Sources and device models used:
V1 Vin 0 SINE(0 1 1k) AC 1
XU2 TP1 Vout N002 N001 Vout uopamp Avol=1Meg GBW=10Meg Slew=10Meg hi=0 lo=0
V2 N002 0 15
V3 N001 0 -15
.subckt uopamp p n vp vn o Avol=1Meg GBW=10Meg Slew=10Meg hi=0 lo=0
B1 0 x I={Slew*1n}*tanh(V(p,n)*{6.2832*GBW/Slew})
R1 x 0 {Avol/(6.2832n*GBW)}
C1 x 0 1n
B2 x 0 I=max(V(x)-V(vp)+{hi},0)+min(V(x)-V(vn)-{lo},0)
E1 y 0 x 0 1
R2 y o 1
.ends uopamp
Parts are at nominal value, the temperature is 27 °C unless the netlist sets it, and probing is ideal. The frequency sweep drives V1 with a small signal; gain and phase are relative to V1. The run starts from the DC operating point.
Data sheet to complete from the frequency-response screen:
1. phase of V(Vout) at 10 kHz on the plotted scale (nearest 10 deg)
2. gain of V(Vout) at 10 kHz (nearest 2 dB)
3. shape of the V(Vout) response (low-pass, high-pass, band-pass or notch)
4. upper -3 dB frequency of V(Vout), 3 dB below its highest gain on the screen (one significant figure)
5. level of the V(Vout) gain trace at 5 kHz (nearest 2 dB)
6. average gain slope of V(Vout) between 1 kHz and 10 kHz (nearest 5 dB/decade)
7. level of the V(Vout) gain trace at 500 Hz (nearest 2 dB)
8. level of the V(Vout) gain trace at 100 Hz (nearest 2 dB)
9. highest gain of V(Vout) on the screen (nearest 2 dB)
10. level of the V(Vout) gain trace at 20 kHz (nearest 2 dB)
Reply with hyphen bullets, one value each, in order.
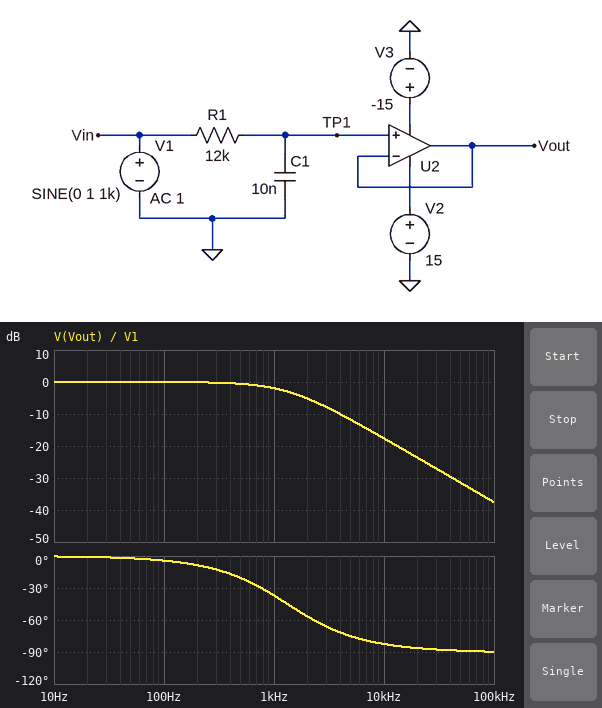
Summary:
- -80 deg
- -18 dB
- low-pass
- 1 kHz
- -12 dB
- -15 dB/decade
- 0 dB
- 0 dB
- 0 dB
- -24 dB
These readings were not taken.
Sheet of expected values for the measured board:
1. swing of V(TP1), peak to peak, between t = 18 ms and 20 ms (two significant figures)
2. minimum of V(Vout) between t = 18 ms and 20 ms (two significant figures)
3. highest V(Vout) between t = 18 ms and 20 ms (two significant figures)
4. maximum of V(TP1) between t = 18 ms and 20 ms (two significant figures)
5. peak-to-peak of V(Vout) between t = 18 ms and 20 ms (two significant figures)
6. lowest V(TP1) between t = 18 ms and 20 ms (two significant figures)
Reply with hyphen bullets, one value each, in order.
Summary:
- 1.6 V
- -800 mV
- 800 mV
- 800 mV
- 1.6 V
- -800 mV
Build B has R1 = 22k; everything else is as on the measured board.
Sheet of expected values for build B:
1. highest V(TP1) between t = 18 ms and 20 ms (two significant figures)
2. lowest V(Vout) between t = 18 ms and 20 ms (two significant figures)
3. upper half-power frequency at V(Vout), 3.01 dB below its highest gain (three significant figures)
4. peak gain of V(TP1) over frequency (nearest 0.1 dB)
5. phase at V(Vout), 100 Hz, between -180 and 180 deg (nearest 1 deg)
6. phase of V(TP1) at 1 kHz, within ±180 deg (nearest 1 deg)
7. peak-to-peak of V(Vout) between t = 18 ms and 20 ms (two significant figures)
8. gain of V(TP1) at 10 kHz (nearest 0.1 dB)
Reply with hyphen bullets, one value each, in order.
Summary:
- 590 mV
- -590 mV
- 723 Hz
- 0 dB
- -8 deg
- -54 deg
- 1.2 V
- -22.8 dB
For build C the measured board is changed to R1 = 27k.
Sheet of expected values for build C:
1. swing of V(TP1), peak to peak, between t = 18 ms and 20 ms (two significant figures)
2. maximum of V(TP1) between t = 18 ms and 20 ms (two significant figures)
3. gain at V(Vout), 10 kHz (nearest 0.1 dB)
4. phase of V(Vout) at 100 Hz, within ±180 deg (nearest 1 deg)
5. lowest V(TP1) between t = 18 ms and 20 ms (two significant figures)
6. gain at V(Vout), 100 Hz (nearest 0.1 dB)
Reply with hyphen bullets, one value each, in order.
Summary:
- 1.0 V
- 510 mV
- -24.6 dB
- -10 deg
- -510 mV
- -0.1 dB
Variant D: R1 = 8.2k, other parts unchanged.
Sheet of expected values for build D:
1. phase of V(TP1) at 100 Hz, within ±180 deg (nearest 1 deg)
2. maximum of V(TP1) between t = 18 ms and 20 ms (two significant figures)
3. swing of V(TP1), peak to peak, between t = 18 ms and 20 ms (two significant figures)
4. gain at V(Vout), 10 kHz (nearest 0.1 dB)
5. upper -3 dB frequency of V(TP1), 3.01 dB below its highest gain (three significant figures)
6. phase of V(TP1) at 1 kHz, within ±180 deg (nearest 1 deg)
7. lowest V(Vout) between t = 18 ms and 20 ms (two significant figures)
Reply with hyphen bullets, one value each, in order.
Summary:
- -3 deg
- 890 mV
- 1.8 V
- -14.4 dB
- 1.94 kHz
- -27 deg
- -890 mV
